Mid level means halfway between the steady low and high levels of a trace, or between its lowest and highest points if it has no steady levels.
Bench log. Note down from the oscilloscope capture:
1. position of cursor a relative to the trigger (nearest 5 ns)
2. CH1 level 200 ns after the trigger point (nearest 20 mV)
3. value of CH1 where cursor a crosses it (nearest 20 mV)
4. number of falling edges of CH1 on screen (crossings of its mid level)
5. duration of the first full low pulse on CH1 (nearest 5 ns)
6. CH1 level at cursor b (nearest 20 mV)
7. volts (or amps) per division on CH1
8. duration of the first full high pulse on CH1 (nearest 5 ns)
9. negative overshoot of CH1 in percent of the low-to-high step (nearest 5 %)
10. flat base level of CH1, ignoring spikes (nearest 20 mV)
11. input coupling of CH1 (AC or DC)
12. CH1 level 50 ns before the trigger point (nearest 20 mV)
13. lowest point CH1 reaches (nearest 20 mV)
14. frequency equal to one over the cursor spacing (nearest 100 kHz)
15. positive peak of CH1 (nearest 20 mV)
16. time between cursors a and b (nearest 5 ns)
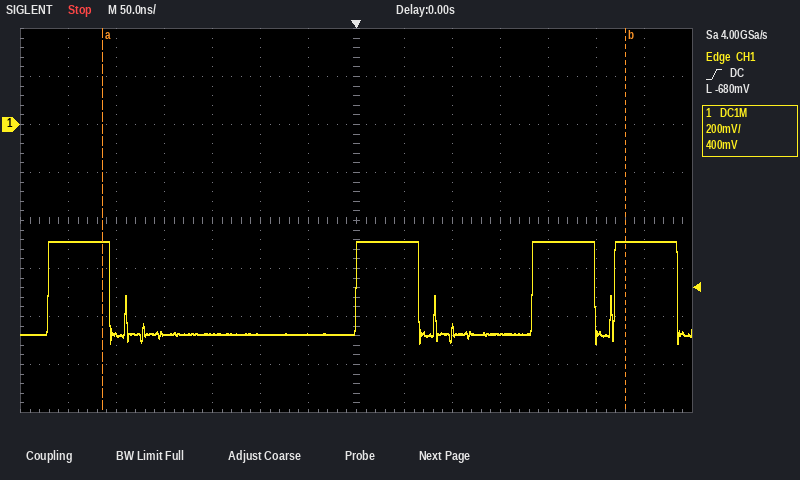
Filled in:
-265 ns
-480 mV
-480 mV
4
255 ns
-480 mV
200 mV
65 ns
10 %
-880 mV
DC
-880 mV
-920 mV
1.8 MHz
-480 mV
545 ns
